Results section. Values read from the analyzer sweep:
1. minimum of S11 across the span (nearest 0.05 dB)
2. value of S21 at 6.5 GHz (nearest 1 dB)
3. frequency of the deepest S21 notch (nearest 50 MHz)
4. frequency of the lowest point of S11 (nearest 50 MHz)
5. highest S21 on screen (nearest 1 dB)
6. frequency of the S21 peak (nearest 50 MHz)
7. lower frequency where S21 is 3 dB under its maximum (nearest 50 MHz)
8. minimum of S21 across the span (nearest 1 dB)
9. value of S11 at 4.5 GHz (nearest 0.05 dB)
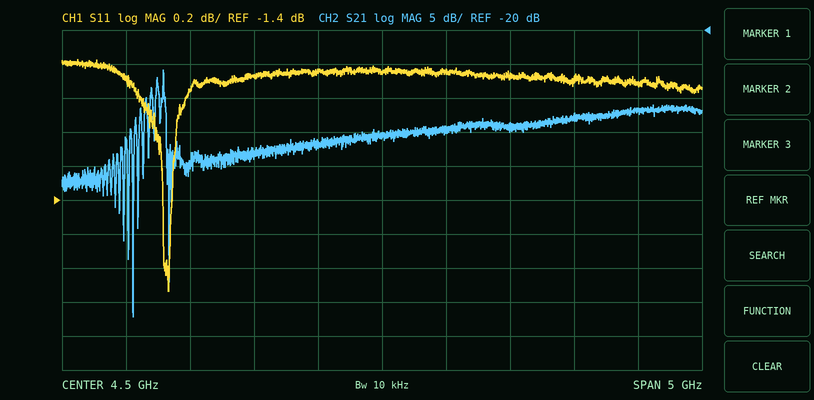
-1.95 dB
-32 dB
2.55 GHz
2.85 GHz
-26 dB
2.80 GHz
2.80 GHz
-62 dB
-0.65 dB
